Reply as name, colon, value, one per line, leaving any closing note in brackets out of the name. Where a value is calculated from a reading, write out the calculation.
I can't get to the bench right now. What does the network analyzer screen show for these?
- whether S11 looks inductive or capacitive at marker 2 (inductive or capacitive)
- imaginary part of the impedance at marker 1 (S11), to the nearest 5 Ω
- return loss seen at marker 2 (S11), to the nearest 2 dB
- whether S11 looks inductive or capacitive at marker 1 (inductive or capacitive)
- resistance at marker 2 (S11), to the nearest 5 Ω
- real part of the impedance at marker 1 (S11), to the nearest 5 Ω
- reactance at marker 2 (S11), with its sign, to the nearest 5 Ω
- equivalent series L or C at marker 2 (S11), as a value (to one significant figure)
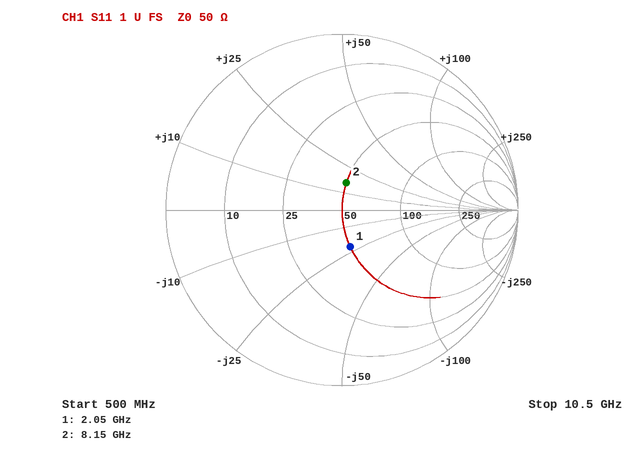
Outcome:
whether S11 looks inductive or capacitive at marker 2: inductive
imaginary part of the impedance at marker 1 (S11), to the nearest 5 Ω: -20 Ω
return loss seen at marker 2 (S11), to the nearest 2 dB: 16 dB
whether S11 looks inductive or capacitive at marker 1: capacitive
resistance at marker 2 (S11), to the nearest 5 Ω: 50 Ω
real part of the impedance at marker 1 (S11), to the nearest 5 Ω: 50 Ω
reactance at marker 2 (S11), with its sign, to the nearest 5 Ω: +15 Ω
equivalent series L or C at marker 2 (S11), as a value: L = 15 Ω/(2π × 8.15 GHz) ≈ 293 pH, so 300 pH to one significant figure
